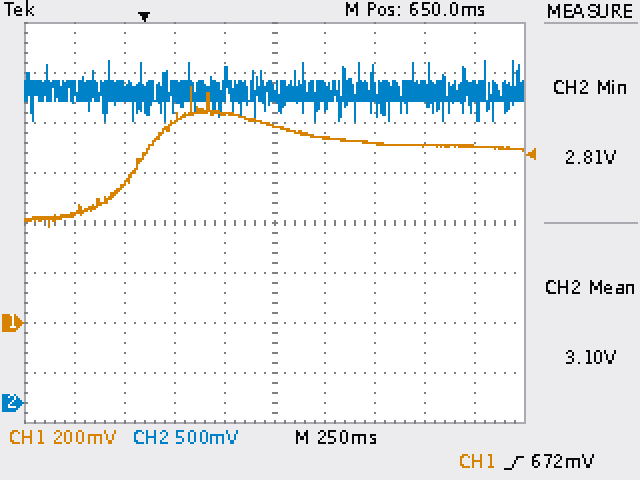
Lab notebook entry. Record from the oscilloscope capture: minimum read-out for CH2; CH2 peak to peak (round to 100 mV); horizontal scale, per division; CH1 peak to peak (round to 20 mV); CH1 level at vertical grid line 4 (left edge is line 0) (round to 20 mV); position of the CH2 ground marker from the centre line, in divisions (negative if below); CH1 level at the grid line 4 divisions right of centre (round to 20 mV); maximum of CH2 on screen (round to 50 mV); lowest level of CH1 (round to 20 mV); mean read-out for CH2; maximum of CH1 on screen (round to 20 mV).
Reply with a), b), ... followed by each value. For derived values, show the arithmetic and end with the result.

a) 2.81 V
b) 600 mV
c) 250 ms
d) 940 mV − (380 mV) = 560 mV
e) 840 mV
f) -3.6 div
g) 700 mV
h) 3.40 V
i) 380 mV
j) 3.10 V
k) 940 mV
